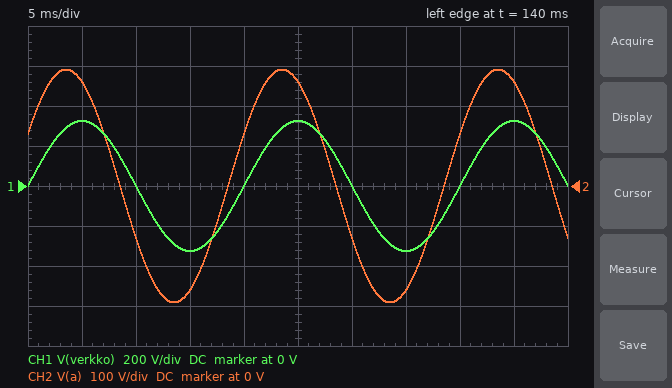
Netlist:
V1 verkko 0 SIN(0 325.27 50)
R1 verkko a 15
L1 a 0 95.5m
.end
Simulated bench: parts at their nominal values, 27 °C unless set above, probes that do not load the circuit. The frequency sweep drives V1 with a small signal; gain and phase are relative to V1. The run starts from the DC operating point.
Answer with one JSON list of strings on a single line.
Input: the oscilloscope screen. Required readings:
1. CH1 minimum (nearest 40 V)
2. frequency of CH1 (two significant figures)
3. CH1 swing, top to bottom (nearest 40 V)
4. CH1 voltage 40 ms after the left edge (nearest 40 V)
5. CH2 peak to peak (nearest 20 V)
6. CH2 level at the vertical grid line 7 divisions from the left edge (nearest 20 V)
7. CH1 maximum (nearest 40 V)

["-320 V", "50 Hz", "640 V", "0 V", "580 V", "-260 V", "320 V"]
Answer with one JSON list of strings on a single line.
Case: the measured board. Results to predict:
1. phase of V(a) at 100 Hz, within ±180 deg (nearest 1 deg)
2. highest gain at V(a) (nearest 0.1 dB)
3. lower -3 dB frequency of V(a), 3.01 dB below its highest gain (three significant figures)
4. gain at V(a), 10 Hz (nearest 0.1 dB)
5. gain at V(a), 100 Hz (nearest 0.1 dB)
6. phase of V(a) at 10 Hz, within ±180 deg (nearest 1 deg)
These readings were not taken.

["14 deg", "0 dB", "25.0 Hz", "-8.6 dB", "-0.3 dB", "68 deg"]
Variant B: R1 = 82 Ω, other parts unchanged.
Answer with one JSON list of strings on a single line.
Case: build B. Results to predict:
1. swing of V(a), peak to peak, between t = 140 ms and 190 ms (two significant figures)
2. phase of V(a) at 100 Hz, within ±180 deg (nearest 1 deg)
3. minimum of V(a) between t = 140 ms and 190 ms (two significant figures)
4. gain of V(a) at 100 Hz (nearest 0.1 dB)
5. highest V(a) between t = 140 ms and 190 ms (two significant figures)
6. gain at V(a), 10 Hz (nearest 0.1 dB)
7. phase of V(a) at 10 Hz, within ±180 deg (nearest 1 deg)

["220 V", "54 deg", "-110 V", "-4.6 dB", "110 V", "-22.7 dB", "86 deg"]
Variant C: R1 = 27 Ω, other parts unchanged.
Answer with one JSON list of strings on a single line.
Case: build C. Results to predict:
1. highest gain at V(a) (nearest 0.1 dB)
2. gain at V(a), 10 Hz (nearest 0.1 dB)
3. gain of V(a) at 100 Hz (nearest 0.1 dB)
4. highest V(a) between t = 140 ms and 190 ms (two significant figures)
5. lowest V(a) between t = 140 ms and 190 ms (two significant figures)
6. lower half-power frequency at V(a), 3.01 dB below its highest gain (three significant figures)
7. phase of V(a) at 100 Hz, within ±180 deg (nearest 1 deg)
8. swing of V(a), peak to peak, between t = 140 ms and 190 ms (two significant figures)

["0 dB", "-13.3 dB", "-0.8 dB", "240 V", "-240 V", "45.0 Hz", "24 deg", "480 V"]
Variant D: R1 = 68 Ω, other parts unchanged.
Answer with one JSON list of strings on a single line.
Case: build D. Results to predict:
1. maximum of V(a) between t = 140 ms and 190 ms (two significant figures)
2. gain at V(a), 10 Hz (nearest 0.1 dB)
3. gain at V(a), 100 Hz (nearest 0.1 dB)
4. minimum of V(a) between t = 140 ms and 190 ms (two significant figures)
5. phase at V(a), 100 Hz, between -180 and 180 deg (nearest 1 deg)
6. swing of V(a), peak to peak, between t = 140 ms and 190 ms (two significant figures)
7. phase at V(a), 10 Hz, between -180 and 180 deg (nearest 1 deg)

["130 V", "-21.1 dB", "-3.6 dB", "-130 V", "49 deg", "260 V", "85 deg"]
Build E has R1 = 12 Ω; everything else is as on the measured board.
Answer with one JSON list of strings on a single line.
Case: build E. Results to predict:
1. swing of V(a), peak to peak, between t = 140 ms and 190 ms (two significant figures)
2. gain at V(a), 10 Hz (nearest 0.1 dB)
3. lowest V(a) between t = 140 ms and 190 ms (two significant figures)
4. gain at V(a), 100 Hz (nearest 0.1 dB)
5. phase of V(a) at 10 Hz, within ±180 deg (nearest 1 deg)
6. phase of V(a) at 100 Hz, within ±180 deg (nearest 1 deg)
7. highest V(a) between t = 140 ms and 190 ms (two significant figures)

["600 V", "-7.0 dB", "-300 V", "-0.2 dB", "63 deg", "11 deg", "300 V"]
